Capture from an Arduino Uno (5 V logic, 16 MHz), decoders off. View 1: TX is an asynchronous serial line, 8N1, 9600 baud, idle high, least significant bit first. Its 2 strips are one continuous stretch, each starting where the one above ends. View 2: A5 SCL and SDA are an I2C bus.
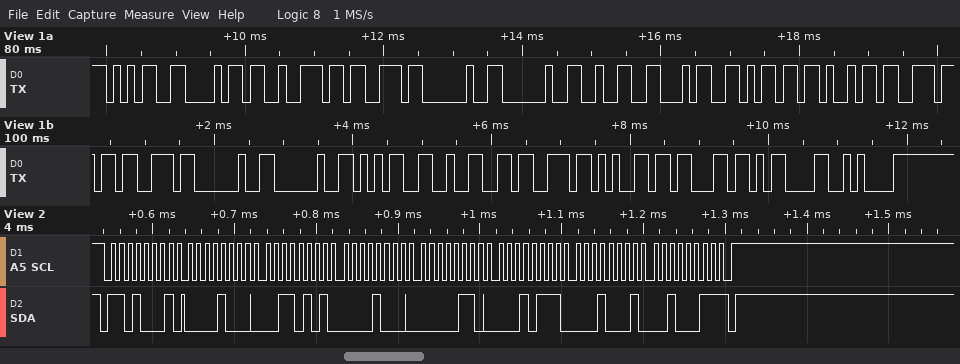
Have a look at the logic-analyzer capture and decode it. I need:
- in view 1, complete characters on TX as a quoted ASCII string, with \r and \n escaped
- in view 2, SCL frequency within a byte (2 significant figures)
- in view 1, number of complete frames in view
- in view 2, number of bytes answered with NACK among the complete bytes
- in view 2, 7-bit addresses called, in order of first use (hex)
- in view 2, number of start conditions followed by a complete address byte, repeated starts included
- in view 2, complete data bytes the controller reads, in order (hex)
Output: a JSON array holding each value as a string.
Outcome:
["\"5hrs  24mins  52sec\\r\\n\"", "100 kHz", "21", "1", "0x68", "1", "08 35 08 06 17 11 23"]
